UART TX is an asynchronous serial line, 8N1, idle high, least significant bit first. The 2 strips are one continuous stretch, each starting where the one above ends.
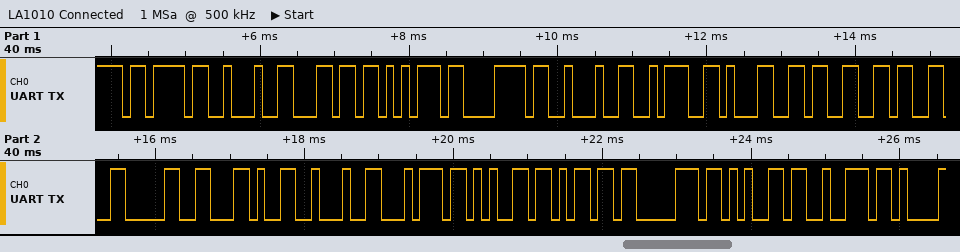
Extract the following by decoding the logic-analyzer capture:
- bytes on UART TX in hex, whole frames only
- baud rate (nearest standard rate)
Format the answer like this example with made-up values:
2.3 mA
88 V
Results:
0x7B 0x22 0x6C 0x75 0x78 0x22 0x3A 0x31 0x33 0x33 0x30 0x2C 0x22 0x74 0x65 0x6D 0x70 0x65 0x72
9600 baud
